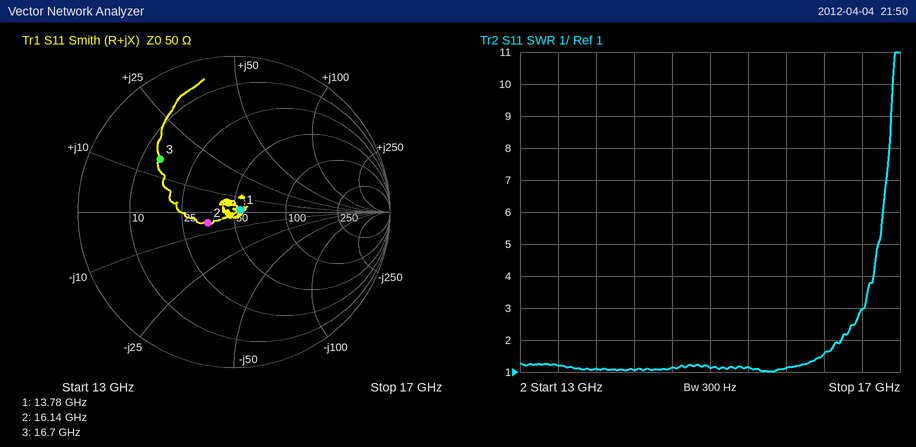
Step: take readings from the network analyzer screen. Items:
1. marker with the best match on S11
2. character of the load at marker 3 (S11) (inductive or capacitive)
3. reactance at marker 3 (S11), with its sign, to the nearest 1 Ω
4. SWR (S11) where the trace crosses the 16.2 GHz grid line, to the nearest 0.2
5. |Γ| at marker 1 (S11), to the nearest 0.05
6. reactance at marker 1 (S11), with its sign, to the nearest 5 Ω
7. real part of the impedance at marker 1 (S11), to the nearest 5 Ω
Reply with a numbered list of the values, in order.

1. marker 1
2. inductive
3. +15 Ω
4. 1.6
5. 0.05
6. 0 Ω
7. 55 Ω
